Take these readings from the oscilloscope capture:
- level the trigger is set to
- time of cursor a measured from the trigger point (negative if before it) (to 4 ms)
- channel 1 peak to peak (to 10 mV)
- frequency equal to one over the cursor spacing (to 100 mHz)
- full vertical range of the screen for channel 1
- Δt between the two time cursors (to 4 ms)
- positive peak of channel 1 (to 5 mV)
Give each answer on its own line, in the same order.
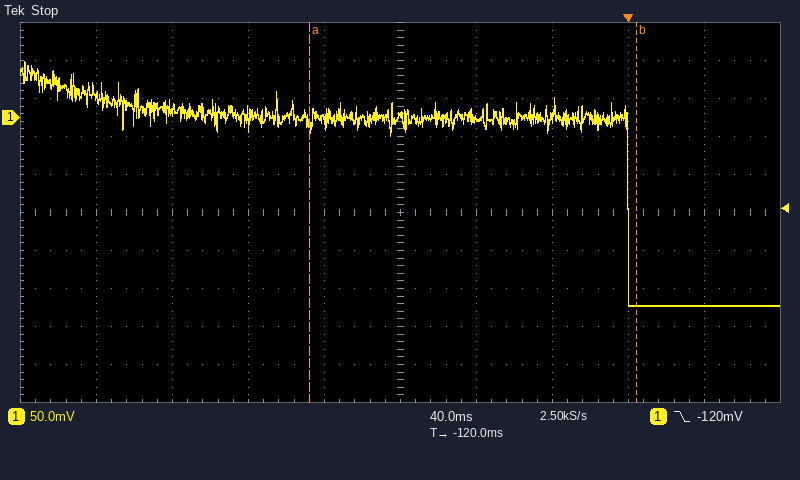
-120 mV
-168 ms
320 mV
5.8 Hz
500 mV
172 ms
75 mV
